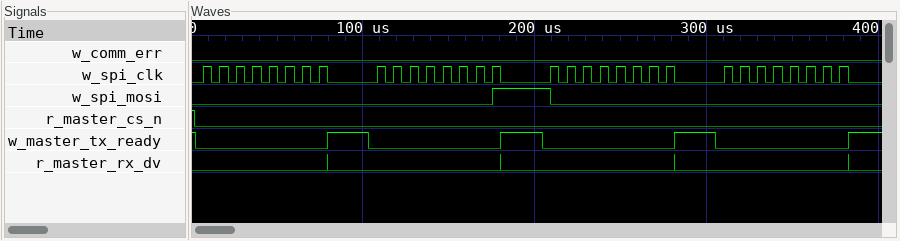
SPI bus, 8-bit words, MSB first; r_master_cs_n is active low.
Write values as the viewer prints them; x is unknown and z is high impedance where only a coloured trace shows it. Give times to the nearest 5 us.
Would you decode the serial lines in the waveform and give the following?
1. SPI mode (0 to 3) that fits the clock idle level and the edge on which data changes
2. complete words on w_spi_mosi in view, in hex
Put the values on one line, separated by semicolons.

1; 00, 01, 00, 00
